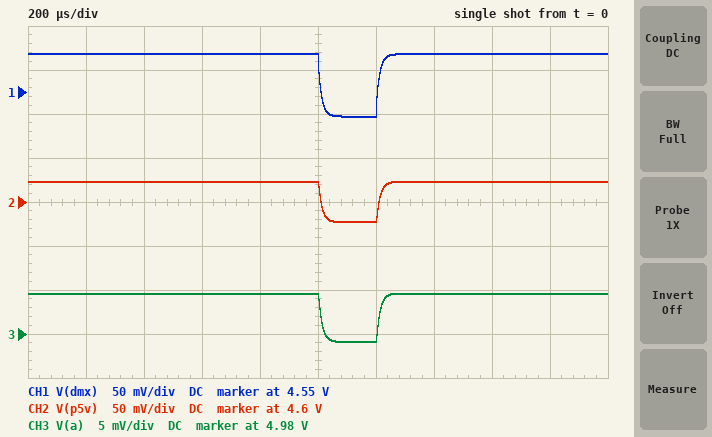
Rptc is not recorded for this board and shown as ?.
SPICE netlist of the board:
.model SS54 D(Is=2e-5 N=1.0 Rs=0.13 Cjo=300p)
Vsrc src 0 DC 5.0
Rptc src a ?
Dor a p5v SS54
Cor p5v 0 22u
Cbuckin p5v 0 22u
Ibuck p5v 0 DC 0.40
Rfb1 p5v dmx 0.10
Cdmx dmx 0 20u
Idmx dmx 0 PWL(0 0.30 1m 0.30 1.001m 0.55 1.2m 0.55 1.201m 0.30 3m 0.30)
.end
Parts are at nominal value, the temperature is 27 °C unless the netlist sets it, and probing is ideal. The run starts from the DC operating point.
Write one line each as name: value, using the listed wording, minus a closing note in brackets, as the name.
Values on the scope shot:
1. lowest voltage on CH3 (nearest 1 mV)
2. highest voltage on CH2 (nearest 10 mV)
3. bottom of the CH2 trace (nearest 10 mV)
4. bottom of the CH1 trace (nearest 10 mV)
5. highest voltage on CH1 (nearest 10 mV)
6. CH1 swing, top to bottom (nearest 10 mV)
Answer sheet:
lowest voltage on CH3: 4.979 V
highest voltage on CH2: 4.62 V
bottom of the CH2 trace: 4.58 V
bottom of the CH1 trace: 4.52 V
highest voltage on CH1: 4.59 V
CH1 swing, top to bottom: 70 mV
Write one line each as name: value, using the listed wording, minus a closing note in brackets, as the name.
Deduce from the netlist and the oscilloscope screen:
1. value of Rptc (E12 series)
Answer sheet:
value of Rptc: 0.022 Ω
